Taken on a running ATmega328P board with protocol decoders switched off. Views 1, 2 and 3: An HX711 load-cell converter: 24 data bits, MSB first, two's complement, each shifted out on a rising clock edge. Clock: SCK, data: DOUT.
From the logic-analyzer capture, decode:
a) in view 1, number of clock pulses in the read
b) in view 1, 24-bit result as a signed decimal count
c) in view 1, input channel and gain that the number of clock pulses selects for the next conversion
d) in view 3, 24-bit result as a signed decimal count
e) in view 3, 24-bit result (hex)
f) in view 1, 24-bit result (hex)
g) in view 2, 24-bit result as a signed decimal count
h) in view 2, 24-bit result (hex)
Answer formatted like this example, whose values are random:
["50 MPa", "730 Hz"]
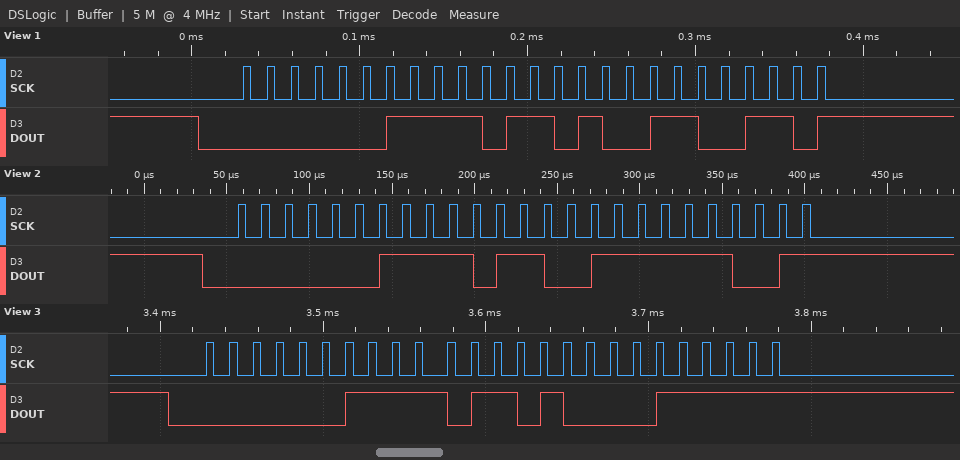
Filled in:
["25", "252518", "channel A, gain 128", "252447", "0x03DA1F", "0x03DA66", "252409", "0x03D9F9"]
